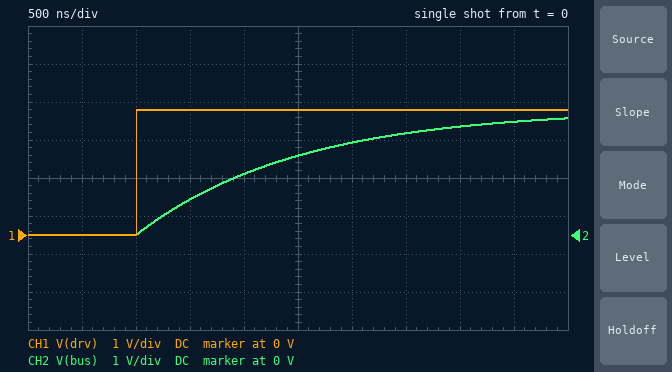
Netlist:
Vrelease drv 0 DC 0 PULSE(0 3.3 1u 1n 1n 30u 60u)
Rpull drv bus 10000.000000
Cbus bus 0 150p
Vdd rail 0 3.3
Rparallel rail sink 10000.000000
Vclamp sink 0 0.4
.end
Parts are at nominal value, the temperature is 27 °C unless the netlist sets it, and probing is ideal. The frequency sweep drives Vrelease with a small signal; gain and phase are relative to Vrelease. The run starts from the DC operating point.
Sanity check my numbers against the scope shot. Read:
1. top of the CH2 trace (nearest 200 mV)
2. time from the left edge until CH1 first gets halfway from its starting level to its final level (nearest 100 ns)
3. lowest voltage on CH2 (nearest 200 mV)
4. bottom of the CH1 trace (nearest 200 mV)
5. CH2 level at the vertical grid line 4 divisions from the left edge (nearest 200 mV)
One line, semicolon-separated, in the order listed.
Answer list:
3.0 V; 1.0 µs; 0 V; 0 V; 1.6 V
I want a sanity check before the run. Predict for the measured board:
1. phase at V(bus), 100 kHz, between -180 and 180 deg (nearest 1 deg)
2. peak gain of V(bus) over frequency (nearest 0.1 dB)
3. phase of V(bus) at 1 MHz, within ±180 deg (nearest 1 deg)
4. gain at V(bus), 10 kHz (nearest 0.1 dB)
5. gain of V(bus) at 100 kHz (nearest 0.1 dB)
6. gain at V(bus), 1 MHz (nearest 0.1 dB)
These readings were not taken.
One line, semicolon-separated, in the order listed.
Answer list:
-43 deg; 0 dB; -84 deg; 0 dB; -2.8 dB; -19.5 dB
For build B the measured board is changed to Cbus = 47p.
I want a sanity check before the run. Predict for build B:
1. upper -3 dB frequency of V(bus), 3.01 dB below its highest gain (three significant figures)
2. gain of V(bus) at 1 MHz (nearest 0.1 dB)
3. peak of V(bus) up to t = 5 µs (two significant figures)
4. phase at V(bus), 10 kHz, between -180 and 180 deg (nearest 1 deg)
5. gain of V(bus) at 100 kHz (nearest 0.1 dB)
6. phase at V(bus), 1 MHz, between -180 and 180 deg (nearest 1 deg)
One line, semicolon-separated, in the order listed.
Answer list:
339 kHz; -9.9 dB; 3.3 V; -2 deg; -0.4 dB; -71 deg
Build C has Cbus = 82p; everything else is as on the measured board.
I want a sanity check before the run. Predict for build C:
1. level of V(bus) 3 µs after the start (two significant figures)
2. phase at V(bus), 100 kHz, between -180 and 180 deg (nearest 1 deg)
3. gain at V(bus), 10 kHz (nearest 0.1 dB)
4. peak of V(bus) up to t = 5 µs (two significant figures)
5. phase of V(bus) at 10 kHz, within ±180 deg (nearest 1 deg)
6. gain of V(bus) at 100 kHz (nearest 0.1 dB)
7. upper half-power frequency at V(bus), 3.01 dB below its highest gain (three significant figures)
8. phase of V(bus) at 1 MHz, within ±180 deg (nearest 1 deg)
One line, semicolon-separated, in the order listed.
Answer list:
3.0 V; -27 deg; 0 dB; 3.3 V; -3 deg; -1.0 dB; 194 kHz; -79 deg
